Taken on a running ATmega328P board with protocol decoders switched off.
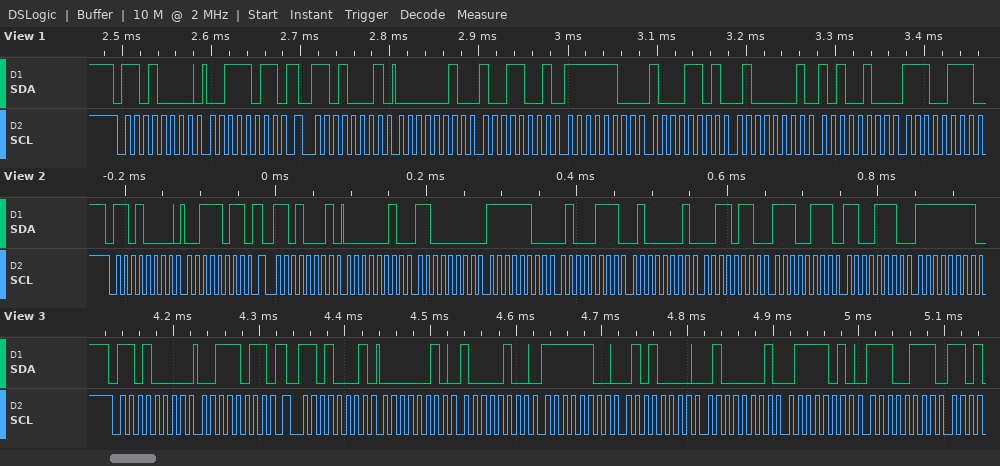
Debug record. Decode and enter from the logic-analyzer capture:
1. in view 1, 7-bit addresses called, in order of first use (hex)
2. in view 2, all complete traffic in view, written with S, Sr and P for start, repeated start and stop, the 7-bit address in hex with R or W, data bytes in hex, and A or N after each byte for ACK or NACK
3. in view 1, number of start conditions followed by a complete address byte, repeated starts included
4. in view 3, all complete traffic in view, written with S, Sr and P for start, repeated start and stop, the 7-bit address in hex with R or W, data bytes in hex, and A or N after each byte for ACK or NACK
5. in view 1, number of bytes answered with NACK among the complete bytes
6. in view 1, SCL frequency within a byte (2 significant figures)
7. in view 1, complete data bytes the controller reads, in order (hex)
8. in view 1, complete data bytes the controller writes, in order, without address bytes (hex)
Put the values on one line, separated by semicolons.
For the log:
0x68; S 68W A 3B A Sr 68R A 02 A C0 A FC A 47 A 41 A 36 A E7 A CE A FF A; 2; S 68W A 3B A Sr 68R A 02 A 84 A FC A 50 A 41 A 7A A E7 A; 0; 100 kHz; 02 99 FC 8D 41 A4 E7; 3B
